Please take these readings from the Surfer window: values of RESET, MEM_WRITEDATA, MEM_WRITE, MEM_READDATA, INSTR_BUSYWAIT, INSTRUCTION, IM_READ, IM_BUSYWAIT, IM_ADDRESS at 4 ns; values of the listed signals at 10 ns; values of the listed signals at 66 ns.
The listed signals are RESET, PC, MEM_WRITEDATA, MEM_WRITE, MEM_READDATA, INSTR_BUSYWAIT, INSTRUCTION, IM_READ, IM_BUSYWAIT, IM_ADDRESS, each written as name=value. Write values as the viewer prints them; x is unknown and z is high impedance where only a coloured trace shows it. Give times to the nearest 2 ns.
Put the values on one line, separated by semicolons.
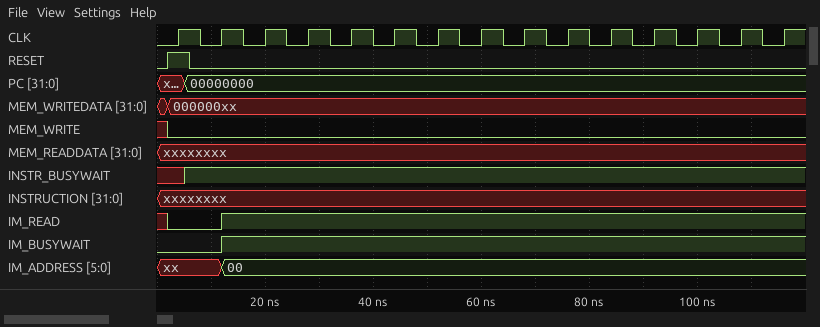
RESET=1, MEM_WRITEDATA=000000xx, MEM_WRITE=0, MEM_READDATA=xxxxxxxx, INSTR_BUSYWAIT=x, INSTRUCTION=xxxxxxxx, IM_READ=0, IM_BUSYWAIT=0, IM_ADDRESS=xx; RESET=0, PC=00000000, MEM_WRITEDATA=000000xx, MEM_WRITE=0, MEM_READDATA=xxxxxxxx, INSTR_BUSYWAIT=1, INSTRUCTION=xxxxxxxx, IM_READ=0, IM_BUSYWAIT=0, IM_ADDRESS=xx; RESET=0, PC=00000000, MEM_WRITEDATA=000000xx, MEM_WRITE=0, MEM_READDATA=xxxxxxxx, INSTR_BUSYWAIT=1, INSTRUCTION=xxxxxxxx, IM_READ=1, IM_BUSYWAIT=1, IM_ADDRESS=00
